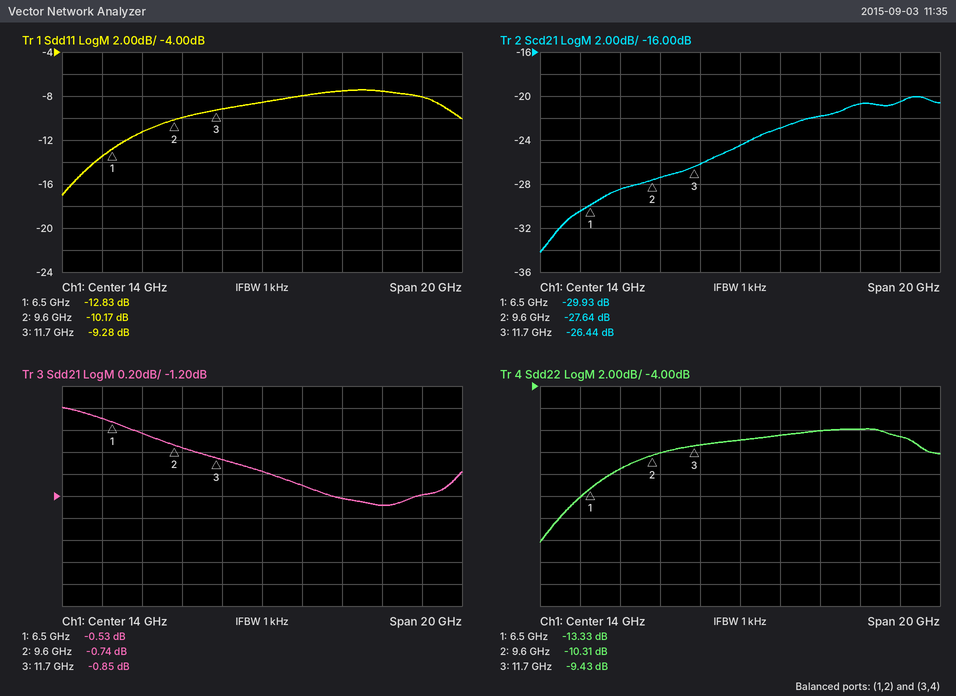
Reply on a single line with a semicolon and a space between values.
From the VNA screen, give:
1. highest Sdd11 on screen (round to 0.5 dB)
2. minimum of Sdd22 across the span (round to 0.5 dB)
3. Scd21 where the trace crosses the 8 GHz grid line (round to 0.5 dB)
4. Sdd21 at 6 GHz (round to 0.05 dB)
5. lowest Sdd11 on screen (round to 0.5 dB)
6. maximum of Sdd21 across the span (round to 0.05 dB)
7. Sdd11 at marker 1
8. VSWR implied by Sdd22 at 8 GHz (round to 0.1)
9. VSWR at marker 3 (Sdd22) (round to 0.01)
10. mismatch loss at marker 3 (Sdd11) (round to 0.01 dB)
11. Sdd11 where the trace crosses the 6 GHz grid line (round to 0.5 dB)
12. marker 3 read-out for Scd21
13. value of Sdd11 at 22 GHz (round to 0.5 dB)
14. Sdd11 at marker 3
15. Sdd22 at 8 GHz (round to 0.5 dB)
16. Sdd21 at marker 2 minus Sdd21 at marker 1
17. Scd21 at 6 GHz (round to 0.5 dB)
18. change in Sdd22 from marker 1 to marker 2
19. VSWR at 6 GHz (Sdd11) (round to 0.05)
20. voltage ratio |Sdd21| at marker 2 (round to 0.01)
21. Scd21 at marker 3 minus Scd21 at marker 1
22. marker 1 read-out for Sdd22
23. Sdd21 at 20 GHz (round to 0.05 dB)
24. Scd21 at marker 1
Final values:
-7.5 dB; -18.0 dB; -28.5 dB; -0.50 dB; -17.0 dB; -0.40 dB; -12.83 dB; 1.7; 2.02; 0.55 dB; -13.5 dB; -26.44 dB; -8.0 dB; -9.28 dB; -11.5 dB; -0.21 dB; -30.5 dB; 3.02 dB; 1.55; 0.92; 3.49 dB; -13.33 dB; -1.30 dB; -29.93 dB
